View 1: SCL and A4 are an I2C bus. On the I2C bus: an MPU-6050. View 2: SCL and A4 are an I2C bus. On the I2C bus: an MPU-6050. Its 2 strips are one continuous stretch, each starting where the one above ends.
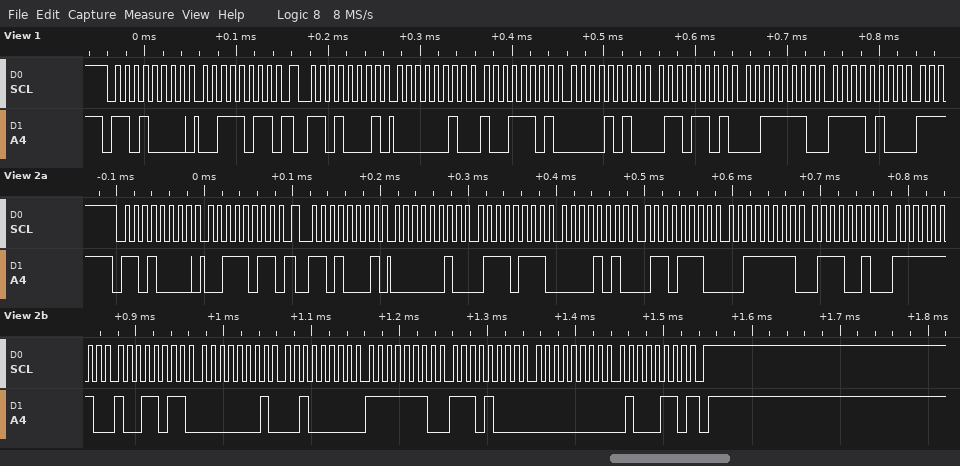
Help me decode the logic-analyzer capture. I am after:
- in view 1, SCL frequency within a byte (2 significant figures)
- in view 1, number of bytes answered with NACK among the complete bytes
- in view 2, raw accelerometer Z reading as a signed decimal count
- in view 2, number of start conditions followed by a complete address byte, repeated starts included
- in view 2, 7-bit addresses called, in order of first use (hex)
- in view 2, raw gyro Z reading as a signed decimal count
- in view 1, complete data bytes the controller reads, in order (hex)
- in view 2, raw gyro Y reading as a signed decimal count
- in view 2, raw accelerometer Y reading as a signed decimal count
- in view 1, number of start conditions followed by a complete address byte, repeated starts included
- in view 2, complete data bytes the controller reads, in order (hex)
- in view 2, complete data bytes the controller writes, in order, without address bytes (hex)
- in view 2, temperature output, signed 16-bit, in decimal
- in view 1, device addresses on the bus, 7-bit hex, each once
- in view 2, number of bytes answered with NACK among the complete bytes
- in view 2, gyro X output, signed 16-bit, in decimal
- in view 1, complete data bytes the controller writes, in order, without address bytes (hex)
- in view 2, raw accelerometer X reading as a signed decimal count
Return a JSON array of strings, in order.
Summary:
["100 kHz", "0", "16242", "2", "0x68", "70", "02 9D 0A 6D 3E F4", "-280", "2670", "2", "02 77 0A 6E 3F 72 FE 9B 01 20 FE E8 00 46", "3B", "-357", "0x68", "1", "288", "3B", "631"]
